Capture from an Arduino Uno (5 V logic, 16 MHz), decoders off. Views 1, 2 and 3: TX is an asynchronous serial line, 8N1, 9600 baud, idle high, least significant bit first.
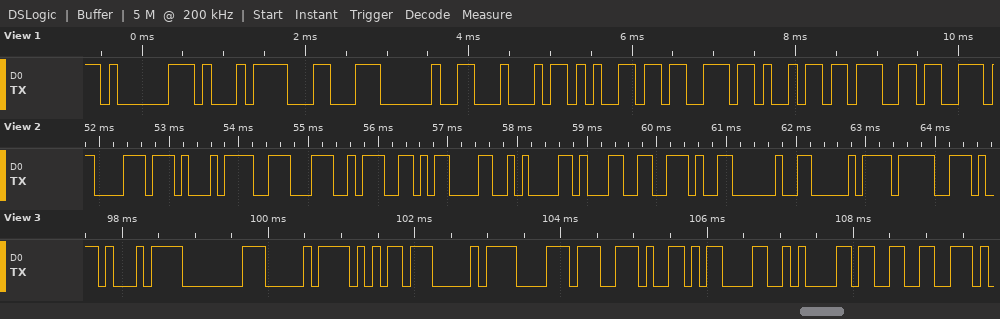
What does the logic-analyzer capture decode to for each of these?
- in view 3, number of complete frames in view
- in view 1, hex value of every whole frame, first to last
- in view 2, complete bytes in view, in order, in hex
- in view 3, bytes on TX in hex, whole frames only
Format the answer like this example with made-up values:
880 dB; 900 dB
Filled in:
10; 81 D1 8C 20 44 65 73 69 67; 0xB8 0xD1 0x8E 0x3A 0x0D 0x0A 0x31 0x2E 0x20 0xD0 0x9F; 0xD1 0x80 0xD0 0xB5 0xD0 0xB8 0x2E 0x0D 0x0A 0x33
